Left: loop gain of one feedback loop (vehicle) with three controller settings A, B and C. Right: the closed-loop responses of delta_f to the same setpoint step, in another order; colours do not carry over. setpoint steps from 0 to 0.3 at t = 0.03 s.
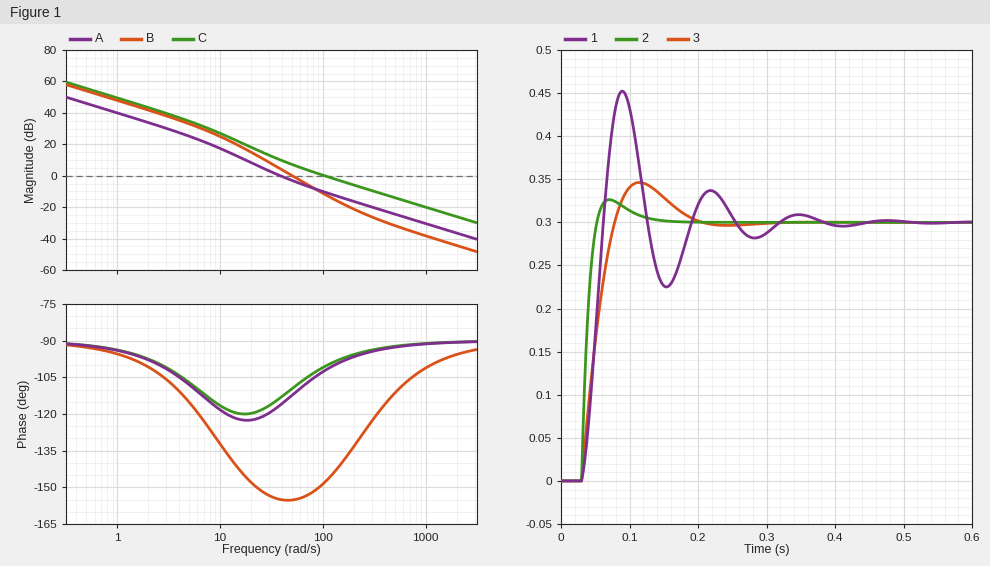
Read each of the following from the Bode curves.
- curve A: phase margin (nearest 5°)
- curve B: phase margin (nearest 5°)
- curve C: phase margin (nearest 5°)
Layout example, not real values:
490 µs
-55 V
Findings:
65°
25°
80°
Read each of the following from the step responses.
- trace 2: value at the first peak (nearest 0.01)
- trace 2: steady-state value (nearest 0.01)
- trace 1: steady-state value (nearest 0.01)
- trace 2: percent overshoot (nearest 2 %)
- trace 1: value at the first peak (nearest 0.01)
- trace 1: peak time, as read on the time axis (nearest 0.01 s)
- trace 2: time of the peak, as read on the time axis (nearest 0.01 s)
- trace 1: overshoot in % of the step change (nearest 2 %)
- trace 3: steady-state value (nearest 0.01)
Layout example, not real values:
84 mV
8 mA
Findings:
0.33
0.30
0.30
8 %
0.45
0.09 s
0.07 s
50 %
0.30
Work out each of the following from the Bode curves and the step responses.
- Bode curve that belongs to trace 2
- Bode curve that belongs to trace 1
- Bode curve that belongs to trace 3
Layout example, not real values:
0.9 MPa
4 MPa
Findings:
C
B
A
